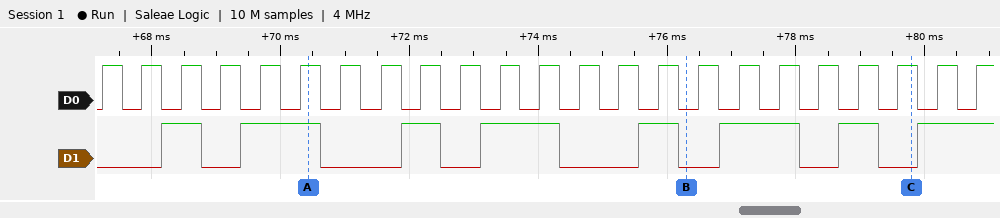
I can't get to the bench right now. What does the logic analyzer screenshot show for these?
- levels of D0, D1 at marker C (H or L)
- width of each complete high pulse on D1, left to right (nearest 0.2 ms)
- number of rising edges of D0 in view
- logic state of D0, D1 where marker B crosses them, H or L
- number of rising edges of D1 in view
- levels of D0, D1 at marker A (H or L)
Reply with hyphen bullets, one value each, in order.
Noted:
- D0=H, D1=L
- 0.6 ms, 1.2 ms, 0.6 ms, 1.2 ms, 0.6 ms, 1.2 ms, 0.6 ms
- 23
- D0=L, D1=L
- 8
- D0=H, D1=H
